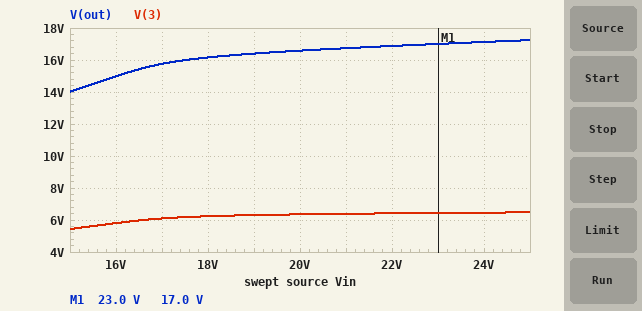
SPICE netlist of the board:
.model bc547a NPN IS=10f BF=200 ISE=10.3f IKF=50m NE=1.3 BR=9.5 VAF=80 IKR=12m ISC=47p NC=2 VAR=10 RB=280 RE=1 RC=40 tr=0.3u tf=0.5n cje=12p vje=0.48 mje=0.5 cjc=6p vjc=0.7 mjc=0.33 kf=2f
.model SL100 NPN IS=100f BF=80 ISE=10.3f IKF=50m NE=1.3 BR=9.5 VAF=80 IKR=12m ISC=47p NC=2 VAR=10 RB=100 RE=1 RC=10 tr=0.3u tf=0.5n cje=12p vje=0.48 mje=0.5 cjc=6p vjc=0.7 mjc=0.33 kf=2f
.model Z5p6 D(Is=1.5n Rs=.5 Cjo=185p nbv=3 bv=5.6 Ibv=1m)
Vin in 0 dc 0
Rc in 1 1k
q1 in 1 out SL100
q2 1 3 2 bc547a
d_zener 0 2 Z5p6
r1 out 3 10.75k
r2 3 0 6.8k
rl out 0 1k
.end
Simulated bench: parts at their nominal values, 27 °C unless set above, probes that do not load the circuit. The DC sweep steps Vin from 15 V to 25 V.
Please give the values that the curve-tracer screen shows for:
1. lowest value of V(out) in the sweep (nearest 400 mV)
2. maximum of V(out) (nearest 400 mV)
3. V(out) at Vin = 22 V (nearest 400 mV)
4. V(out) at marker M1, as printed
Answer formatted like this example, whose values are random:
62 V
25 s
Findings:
14.0 V
17.2 V
16.8 V
17.0 V
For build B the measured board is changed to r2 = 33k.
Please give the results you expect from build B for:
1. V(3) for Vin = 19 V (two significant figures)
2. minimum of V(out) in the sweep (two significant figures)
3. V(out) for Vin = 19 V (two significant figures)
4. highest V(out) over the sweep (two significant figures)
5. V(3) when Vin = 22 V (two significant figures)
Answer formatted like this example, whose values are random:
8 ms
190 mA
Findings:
6.5 V
9.0 V
9.4 V
10 V
6.6 V
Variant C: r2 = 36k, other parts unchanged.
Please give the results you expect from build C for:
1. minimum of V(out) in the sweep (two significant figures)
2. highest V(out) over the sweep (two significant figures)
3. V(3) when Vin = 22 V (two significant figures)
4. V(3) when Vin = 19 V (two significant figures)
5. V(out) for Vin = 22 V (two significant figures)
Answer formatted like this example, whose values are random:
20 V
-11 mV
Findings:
8.8 V
9.9 V
6.6 V
6.5 V
9.6 V
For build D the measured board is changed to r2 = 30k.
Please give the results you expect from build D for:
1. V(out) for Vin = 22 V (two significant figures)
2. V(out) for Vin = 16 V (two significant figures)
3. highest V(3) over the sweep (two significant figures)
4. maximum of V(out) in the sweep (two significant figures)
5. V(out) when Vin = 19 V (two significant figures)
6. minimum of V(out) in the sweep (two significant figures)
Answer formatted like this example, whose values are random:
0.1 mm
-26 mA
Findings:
9.9 V
9.3 V
6.6 V
10 V
9.6 V
9.2 V
